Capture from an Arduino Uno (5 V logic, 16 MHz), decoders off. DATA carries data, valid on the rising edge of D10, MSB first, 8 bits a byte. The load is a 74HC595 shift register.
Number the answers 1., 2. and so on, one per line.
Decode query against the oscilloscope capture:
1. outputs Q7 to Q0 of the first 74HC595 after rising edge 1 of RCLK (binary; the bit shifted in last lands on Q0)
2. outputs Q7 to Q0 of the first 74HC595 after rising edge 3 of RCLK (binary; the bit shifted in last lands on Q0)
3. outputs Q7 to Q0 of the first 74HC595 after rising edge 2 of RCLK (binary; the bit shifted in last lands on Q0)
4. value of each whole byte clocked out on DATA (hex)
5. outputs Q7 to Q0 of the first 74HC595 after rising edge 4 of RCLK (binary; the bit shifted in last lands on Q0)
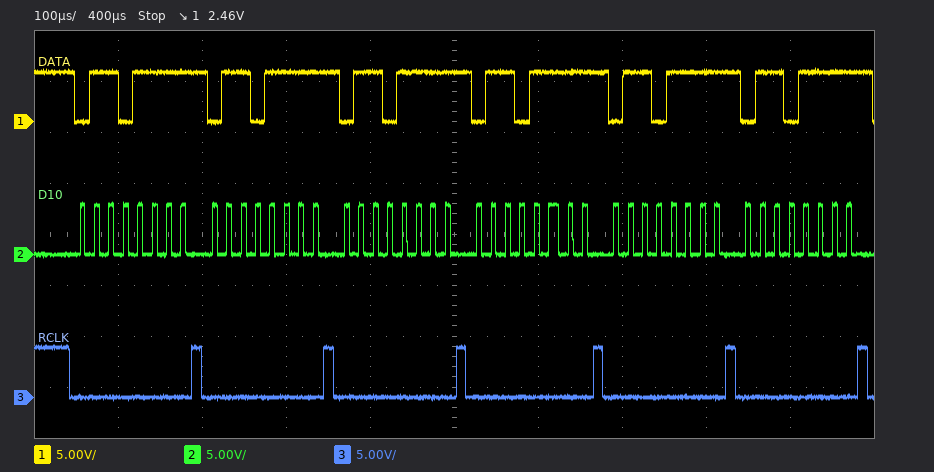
1. 01101111
2. 01101111
3. 01101111
4. 0x6F 0x6F 0x6F 0x6F 0x6F 0x6F
5. 01101111
